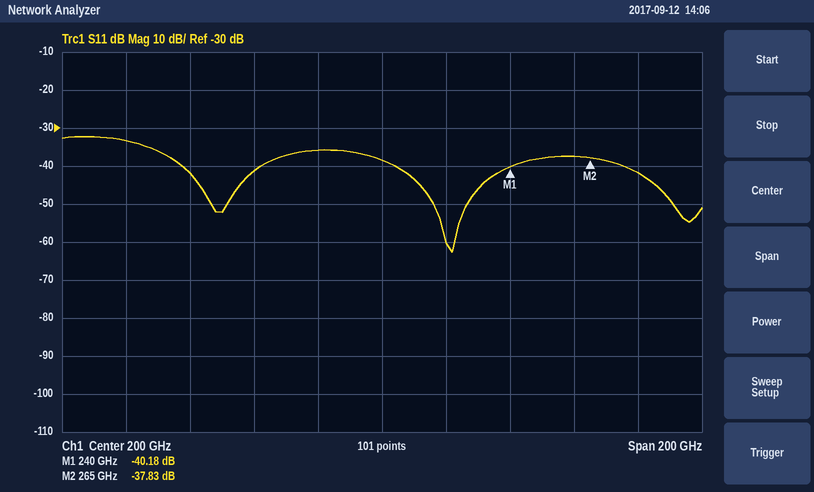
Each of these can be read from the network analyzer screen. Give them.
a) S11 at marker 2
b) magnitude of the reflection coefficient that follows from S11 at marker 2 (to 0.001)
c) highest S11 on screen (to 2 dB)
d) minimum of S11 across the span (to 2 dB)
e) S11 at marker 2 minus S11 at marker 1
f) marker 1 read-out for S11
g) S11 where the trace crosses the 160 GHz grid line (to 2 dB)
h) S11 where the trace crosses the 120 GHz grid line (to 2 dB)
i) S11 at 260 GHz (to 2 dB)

-37.83 dB
0.013
-32 dB
-62 dB
2.35 dB
-40.18 dB
-42 dB
-34 dB
-38 dB
